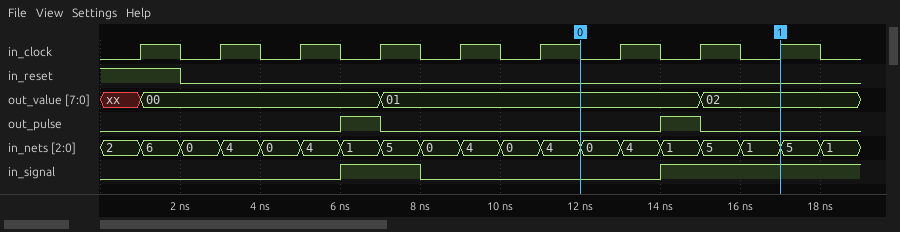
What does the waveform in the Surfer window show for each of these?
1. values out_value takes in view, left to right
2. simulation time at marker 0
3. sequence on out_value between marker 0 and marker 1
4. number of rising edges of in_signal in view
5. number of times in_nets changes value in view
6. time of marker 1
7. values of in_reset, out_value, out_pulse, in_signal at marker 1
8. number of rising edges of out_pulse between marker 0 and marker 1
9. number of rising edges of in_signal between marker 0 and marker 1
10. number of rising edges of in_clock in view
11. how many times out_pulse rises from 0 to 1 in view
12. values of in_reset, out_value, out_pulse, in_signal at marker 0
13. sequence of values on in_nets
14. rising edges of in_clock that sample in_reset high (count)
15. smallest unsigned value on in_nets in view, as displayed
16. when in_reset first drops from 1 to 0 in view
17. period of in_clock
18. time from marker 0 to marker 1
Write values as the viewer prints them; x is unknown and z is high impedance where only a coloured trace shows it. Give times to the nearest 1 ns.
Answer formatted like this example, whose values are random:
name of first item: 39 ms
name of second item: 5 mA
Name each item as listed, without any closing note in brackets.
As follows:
values out_value takes in view, left to right: xx, 00, 01, 02
simulation time at marker 0: 12 ns
sequence on out_value between marker 0 and marker 1: 01, 02
number of rising edges of in_signal in view: 2
number of times in_nets changes value in view: 18
time of marker 1: 17 ns
values of in_reset, out_value, out_pulse, in_signal at marker 1: in_reset=0, out_value=02, out_pulse=0, in_signal=1
number of rising edges of out_pulse between marker 0 and marker 1: 1
number of rising edges of in_signal between marker 0 and marker 1: 1
number of rising edges of in_clock in view: 9
how many times out_pulse rises from 0 to 1 in view: 2
values of in_reset, out_value, out_pulse, in_signal at marker 0: in_reset=0, out_value=01, out_pulse=0, in_signal=0
sequence of values on in_nets: 2, 6, 0, 4, 0, 4, 1, 5, 0, 4, 0, 4, 0, 4, 1, 5, 1, 5, 1
rising edges of in_clock that sample in_reset high: 1
smallest unsigned value on in_nets in view, as displayed: 0
when in_reset first drops from 1 to 0 in view: 2 ns
period of in_clock: 2 ns
time from marker 0 to marker 1: 5 ns
